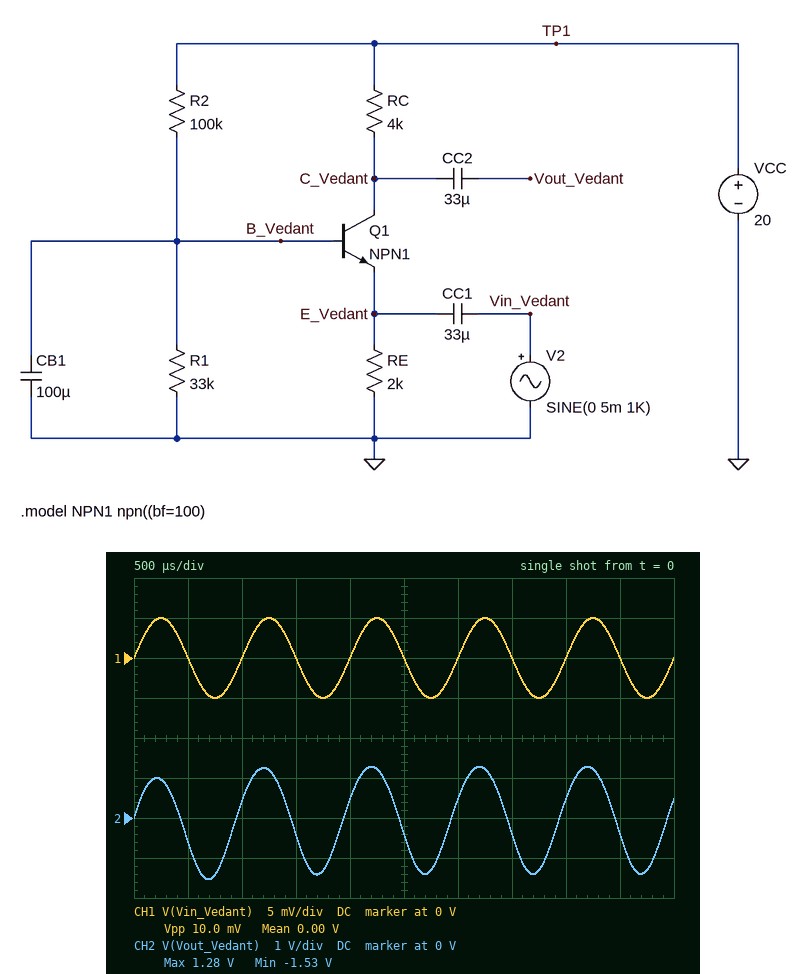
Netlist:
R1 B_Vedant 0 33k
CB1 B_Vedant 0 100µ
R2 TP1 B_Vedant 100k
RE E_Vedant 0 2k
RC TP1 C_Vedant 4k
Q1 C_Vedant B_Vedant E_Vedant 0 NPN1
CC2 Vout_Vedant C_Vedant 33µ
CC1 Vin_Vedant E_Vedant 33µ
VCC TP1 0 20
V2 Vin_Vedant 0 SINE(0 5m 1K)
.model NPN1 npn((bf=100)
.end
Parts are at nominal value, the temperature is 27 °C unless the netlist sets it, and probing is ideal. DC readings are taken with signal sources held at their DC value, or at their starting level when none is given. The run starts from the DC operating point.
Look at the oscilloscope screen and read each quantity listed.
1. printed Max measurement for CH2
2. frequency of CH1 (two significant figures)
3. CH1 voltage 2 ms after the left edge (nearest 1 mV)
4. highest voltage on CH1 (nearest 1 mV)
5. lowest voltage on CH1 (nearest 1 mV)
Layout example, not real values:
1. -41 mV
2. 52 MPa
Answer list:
1. 1.28 V
2. 1.0 kHz
3. 0 V
4. 5 mV
5. -5 mV
